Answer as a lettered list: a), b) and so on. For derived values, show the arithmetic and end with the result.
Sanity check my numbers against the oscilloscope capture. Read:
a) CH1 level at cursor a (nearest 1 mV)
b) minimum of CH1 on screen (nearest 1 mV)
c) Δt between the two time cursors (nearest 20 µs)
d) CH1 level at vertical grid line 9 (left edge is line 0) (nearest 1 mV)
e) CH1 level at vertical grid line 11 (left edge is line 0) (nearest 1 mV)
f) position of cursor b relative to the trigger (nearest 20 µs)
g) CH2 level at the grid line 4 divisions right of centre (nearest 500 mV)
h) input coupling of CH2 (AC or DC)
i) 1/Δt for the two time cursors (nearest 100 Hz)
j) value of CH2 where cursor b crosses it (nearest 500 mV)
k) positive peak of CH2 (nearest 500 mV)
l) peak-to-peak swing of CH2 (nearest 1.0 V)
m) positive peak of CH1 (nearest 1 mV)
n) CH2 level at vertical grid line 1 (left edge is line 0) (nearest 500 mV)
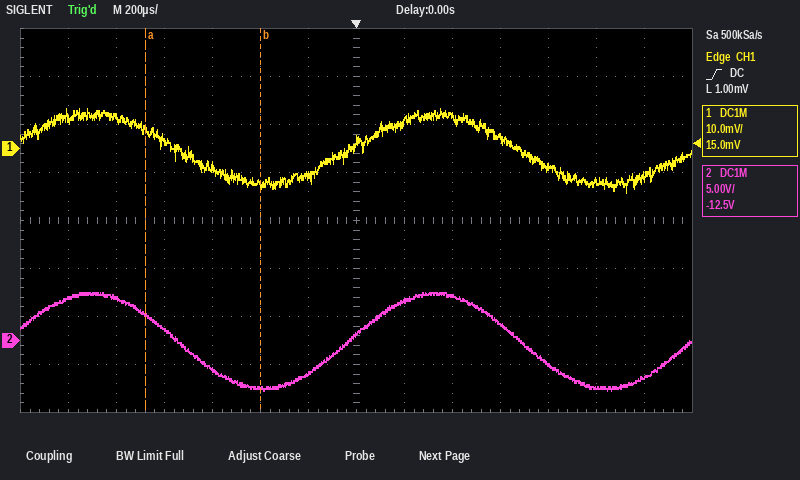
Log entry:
a) 4 mV
b) -9 mV
c) 480 µs
d) 7 mV
e) -4 mV
f) -400 µs
g) -2.5 V
h) DC
i) 1 / 480 µs ≈ 2.1 kHz
j) -5.0 V
k) 5.0 V
l) 10.0 V
m) 8 mV
n) 4.5 V
